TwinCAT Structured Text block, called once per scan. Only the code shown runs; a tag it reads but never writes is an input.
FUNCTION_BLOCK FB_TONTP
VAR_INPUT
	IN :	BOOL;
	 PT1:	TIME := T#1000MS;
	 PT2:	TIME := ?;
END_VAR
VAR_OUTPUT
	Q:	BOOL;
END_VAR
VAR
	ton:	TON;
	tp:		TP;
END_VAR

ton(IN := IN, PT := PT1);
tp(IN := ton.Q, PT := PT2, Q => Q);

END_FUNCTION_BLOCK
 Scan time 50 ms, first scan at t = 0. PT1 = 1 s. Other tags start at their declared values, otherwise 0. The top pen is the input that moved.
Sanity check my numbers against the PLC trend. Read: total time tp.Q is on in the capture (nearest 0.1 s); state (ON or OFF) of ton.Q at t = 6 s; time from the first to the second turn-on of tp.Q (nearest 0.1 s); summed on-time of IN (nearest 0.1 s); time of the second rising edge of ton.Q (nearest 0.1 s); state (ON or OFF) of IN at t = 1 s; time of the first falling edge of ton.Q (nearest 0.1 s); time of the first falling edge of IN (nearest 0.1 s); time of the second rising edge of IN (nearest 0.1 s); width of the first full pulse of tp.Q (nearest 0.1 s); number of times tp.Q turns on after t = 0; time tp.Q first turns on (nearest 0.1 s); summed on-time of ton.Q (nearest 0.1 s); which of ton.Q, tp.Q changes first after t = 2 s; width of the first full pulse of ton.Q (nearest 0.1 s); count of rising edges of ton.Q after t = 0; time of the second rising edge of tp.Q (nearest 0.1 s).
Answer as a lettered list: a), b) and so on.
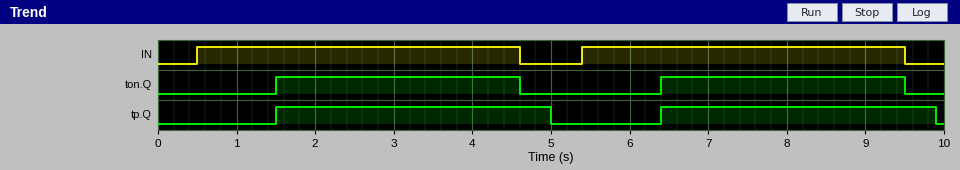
a) 7.0 s
b) OFF
c) 4.9 s
d) 8.2 s
e) 6.4 s
f) ON
g) 4.6 s
h) 4.6 s
i) 5.4 s
j) 3.5 s
k) 2
l) 1.5 s
m) 6.2 s
n) ton.Q
o) 3.1 s
p) 2
q) 6.4 s
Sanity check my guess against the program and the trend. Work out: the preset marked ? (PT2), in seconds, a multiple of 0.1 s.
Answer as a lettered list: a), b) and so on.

a) 3.5 s
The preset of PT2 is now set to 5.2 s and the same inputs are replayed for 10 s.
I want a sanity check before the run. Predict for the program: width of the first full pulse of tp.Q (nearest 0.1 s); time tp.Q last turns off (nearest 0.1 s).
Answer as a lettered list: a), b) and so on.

a) 5.2 s
b) 6.7 s
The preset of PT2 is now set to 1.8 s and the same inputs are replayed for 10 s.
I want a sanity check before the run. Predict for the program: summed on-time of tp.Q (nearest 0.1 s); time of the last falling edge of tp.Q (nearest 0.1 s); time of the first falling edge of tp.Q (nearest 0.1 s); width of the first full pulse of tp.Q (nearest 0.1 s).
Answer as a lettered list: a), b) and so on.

a) 3.6 s
b) 8.2 s
c) 3.3 s
d) 1.8 s
